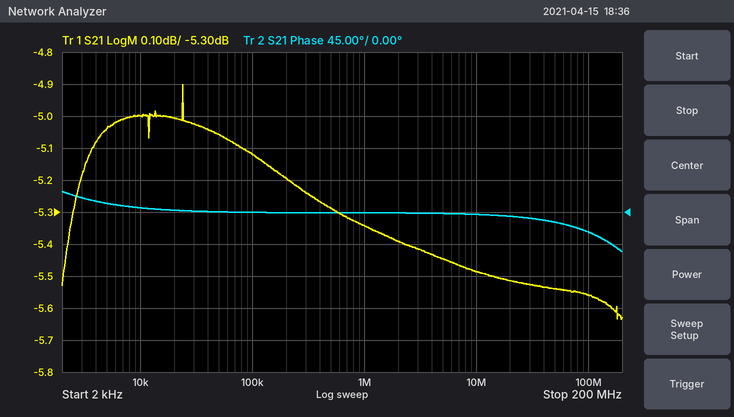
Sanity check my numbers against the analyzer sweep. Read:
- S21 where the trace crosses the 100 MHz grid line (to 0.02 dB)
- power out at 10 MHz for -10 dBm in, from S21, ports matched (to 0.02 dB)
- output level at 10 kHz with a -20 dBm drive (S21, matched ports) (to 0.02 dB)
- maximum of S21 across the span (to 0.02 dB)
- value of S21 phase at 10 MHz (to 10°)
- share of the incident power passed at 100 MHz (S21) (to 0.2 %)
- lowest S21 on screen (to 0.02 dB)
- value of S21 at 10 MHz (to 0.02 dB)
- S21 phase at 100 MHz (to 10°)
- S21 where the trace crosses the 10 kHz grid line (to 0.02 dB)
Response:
-5.56 dB
-15.48 dBm
-25.00 dBm
-4.90 dB
0°
27.8 %
-5.64 dB
-5.48 dB
-30°
-5.00 dB
